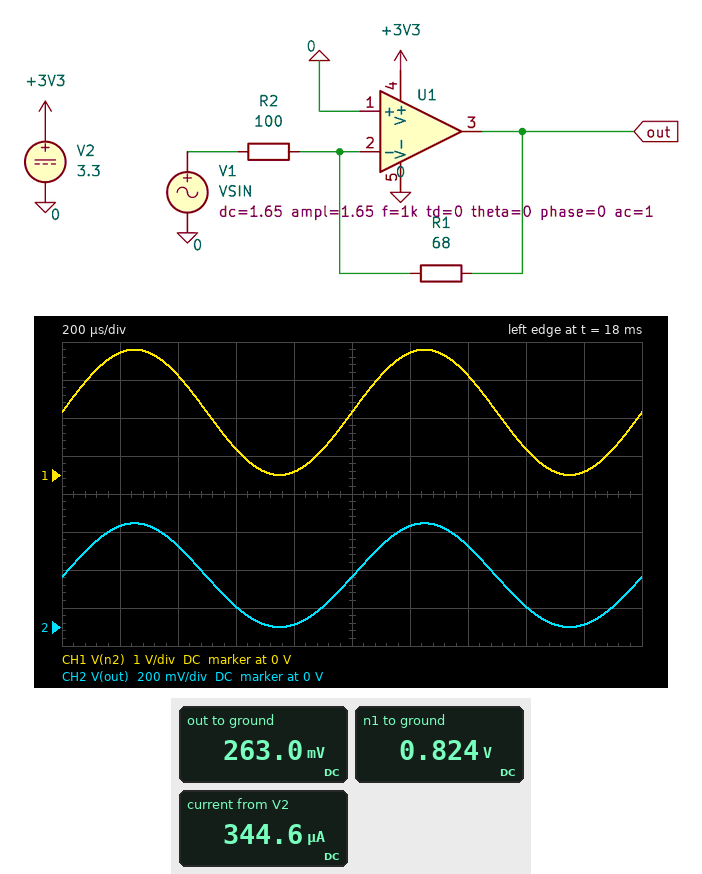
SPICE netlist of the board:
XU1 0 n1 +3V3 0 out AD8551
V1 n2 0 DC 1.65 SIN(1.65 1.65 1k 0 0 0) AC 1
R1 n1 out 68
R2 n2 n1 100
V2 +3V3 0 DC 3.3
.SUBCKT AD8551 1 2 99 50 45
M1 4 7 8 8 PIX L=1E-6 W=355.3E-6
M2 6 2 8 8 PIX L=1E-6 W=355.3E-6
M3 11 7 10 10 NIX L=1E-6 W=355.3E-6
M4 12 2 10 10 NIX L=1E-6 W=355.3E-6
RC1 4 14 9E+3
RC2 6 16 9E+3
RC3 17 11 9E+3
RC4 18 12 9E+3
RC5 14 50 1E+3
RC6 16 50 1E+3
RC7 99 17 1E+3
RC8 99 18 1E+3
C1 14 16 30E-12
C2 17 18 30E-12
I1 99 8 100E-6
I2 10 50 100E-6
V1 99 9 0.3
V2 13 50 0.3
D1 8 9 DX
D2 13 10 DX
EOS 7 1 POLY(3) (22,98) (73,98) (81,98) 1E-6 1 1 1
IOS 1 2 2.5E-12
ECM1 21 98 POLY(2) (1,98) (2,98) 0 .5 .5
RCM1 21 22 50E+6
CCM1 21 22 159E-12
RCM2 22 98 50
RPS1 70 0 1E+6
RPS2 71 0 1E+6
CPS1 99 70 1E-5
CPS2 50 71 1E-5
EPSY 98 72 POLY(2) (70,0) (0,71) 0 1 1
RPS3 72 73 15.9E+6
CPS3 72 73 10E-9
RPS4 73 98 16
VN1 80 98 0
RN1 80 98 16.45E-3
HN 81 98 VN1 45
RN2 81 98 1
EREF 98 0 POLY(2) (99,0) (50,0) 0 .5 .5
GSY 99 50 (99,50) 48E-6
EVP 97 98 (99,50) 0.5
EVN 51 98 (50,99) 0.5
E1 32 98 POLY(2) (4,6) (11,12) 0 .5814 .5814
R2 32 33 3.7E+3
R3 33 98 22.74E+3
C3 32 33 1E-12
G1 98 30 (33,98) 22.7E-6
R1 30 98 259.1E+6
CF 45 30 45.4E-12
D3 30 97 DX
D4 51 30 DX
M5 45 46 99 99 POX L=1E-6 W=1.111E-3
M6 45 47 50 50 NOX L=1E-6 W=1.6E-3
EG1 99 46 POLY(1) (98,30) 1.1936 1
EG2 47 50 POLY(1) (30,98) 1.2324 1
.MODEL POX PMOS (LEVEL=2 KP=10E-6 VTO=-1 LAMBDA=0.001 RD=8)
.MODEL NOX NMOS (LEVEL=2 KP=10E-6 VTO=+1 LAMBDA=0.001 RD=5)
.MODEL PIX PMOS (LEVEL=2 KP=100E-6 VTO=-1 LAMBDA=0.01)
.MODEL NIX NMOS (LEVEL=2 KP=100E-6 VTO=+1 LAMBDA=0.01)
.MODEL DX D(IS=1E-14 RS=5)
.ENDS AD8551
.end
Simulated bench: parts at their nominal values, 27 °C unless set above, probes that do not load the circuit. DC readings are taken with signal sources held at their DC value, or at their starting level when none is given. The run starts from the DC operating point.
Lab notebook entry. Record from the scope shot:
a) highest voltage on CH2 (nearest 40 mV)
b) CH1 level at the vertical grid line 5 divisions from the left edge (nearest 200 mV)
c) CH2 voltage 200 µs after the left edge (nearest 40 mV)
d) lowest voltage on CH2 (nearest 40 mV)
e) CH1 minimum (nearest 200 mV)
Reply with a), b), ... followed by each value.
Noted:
a) 560 mV
b) 1.6 V
c) 520 mV
d) 0 V
e) 0 V
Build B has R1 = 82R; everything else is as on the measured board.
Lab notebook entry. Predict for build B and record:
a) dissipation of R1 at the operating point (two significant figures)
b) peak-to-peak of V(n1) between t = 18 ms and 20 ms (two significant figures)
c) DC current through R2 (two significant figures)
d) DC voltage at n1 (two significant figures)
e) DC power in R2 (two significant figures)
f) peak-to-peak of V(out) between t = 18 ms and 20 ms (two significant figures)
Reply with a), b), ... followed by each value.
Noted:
a) 4.9 mW
b) 1.8 V
c) 7.7 mA
d) 880 mV
e) 6.0 mW
f) 510 mV
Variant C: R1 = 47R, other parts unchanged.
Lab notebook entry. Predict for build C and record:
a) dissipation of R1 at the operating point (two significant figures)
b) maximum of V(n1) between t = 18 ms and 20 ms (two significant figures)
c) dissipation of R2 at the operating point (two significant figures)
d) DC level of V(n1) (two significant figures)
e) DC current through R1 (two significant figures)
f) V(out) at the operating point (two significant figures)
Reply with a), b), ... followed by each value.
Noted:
a) 4.0 mW
b) 1.5 V
c) 8.5 mW
d) 730 mV
e) 9.2 mA
f) 300 mV
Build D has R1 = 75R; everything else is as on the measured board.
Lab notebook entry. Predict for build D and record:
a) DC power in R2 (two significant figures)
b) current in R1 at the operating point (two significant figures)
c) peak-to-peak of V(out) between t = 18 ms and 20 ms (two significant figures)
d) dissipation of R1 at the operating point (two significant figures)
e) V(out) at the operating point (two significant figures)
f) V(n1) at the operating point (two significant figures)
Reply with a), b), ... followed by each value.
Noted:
a) 6.4 mW
b) 8.0 mA
c) 530 mV
d) 4.8 mW
e) 250 mV
f) 850 mV
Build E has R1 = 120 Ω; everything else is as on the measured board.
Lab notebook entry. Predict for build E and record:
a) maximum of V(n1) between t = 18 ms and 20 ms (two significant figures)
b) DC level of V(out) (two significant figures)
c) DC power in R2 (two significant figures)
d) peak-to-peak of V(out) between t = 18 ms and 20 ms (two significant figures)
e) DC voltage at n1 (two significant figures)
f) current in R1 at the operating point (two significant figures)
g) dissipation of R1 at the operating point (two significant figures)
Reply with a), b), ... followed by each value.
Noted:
a) 2.0 V
b) 210 mV
c) 4.3 mW
d) 430 mV
e) 990 mV
f) 6.6 mA
g) 5.2 mW
